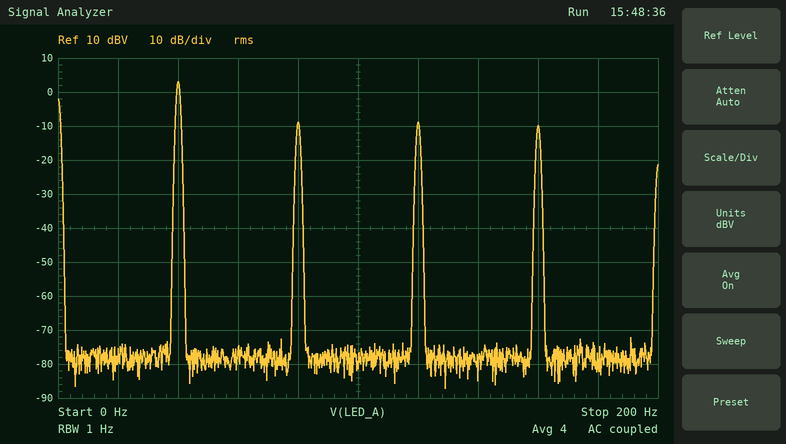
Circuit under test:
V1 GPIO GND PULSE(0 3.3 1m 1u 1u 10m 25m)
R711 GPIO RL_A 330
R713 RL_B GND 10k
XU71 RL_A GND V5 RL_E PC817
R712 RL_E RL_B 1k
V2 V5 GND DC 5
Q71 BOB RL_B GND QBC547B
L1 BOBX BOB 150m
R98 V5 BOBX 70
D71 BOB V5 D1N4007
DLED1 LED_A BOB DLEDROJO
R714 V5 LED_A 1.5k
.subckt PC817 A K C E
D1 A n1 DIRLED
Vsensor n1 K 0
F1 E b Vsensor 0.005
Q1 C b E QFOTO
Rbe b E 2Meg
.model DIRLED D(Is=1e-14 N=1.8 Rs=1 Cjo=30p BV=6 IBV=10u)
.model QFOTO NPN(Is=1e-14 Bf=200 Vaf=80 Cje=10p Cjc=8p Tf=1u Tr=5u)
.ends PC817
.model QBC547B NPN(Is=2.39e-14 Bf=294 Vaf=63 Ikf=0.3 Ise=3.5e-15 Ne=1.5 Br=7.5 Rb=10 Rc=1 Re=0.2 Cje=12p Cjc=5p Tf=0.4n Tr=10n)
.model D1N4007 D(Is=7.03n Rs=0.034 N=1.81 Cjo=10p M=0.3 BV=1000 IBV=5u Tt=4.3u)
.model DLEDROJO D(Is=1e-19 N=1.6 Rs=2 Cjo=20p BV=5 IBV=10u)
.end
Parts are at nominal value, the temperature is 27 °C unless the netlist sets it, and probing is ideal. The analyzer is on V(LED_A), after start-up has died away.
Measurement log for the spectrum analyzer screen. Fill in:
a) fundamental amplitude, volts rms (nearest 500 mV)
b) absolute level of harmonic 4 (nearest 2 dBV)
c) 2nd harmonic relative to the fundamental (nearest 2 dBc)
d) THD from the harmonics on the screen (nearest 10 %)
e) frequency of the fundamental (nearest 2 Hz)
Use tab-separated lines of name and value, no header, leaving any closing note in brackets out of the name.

fundamental amplitude, volts rms	1.5 V
absolute level of harmonic 4	-10 dBV
2nd harmonic relative to the fundamental	-12 dBc
THD from the harmonics on the screen	40 %
frequency of the fundamental	40 Hz
